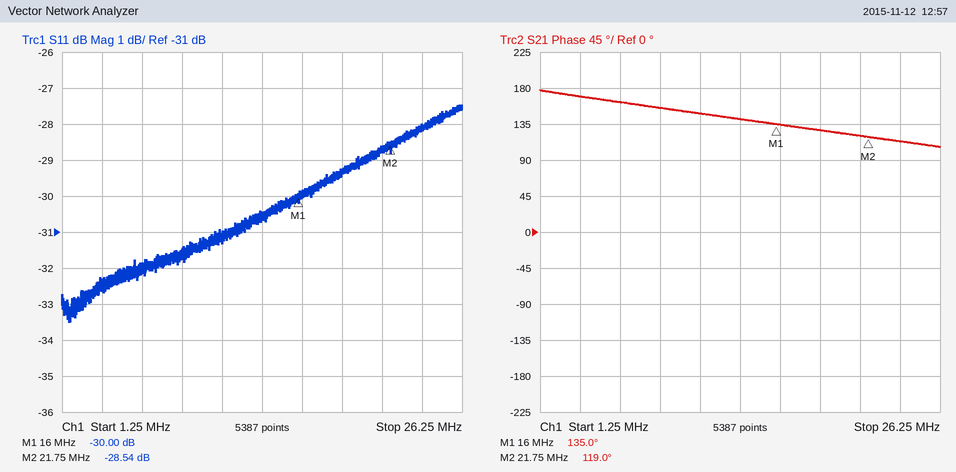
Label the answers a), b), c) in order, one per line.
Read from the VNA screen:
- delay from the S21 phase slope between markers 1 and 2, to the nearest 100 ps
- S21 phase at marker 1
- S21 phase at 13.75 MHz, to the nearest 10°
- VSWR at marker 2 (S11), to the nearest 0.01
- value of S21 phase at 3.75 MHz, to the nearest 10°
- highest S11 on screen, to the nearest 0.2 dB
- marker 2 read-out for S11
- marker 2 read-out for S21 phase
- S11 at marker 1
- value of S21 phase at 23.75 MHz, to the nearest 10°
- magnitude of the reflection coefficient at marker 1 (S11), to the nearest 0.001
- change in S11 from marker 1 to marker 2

a) 7.7 ns
b) 135.0°
c) 140°
d) 1.08
e) 170°
f) -27.4 dB
g) -28.54 dB
h) 119.0°
i) -30.00 dB
j) 110°
k) 0.032
l) 1.46 dB
